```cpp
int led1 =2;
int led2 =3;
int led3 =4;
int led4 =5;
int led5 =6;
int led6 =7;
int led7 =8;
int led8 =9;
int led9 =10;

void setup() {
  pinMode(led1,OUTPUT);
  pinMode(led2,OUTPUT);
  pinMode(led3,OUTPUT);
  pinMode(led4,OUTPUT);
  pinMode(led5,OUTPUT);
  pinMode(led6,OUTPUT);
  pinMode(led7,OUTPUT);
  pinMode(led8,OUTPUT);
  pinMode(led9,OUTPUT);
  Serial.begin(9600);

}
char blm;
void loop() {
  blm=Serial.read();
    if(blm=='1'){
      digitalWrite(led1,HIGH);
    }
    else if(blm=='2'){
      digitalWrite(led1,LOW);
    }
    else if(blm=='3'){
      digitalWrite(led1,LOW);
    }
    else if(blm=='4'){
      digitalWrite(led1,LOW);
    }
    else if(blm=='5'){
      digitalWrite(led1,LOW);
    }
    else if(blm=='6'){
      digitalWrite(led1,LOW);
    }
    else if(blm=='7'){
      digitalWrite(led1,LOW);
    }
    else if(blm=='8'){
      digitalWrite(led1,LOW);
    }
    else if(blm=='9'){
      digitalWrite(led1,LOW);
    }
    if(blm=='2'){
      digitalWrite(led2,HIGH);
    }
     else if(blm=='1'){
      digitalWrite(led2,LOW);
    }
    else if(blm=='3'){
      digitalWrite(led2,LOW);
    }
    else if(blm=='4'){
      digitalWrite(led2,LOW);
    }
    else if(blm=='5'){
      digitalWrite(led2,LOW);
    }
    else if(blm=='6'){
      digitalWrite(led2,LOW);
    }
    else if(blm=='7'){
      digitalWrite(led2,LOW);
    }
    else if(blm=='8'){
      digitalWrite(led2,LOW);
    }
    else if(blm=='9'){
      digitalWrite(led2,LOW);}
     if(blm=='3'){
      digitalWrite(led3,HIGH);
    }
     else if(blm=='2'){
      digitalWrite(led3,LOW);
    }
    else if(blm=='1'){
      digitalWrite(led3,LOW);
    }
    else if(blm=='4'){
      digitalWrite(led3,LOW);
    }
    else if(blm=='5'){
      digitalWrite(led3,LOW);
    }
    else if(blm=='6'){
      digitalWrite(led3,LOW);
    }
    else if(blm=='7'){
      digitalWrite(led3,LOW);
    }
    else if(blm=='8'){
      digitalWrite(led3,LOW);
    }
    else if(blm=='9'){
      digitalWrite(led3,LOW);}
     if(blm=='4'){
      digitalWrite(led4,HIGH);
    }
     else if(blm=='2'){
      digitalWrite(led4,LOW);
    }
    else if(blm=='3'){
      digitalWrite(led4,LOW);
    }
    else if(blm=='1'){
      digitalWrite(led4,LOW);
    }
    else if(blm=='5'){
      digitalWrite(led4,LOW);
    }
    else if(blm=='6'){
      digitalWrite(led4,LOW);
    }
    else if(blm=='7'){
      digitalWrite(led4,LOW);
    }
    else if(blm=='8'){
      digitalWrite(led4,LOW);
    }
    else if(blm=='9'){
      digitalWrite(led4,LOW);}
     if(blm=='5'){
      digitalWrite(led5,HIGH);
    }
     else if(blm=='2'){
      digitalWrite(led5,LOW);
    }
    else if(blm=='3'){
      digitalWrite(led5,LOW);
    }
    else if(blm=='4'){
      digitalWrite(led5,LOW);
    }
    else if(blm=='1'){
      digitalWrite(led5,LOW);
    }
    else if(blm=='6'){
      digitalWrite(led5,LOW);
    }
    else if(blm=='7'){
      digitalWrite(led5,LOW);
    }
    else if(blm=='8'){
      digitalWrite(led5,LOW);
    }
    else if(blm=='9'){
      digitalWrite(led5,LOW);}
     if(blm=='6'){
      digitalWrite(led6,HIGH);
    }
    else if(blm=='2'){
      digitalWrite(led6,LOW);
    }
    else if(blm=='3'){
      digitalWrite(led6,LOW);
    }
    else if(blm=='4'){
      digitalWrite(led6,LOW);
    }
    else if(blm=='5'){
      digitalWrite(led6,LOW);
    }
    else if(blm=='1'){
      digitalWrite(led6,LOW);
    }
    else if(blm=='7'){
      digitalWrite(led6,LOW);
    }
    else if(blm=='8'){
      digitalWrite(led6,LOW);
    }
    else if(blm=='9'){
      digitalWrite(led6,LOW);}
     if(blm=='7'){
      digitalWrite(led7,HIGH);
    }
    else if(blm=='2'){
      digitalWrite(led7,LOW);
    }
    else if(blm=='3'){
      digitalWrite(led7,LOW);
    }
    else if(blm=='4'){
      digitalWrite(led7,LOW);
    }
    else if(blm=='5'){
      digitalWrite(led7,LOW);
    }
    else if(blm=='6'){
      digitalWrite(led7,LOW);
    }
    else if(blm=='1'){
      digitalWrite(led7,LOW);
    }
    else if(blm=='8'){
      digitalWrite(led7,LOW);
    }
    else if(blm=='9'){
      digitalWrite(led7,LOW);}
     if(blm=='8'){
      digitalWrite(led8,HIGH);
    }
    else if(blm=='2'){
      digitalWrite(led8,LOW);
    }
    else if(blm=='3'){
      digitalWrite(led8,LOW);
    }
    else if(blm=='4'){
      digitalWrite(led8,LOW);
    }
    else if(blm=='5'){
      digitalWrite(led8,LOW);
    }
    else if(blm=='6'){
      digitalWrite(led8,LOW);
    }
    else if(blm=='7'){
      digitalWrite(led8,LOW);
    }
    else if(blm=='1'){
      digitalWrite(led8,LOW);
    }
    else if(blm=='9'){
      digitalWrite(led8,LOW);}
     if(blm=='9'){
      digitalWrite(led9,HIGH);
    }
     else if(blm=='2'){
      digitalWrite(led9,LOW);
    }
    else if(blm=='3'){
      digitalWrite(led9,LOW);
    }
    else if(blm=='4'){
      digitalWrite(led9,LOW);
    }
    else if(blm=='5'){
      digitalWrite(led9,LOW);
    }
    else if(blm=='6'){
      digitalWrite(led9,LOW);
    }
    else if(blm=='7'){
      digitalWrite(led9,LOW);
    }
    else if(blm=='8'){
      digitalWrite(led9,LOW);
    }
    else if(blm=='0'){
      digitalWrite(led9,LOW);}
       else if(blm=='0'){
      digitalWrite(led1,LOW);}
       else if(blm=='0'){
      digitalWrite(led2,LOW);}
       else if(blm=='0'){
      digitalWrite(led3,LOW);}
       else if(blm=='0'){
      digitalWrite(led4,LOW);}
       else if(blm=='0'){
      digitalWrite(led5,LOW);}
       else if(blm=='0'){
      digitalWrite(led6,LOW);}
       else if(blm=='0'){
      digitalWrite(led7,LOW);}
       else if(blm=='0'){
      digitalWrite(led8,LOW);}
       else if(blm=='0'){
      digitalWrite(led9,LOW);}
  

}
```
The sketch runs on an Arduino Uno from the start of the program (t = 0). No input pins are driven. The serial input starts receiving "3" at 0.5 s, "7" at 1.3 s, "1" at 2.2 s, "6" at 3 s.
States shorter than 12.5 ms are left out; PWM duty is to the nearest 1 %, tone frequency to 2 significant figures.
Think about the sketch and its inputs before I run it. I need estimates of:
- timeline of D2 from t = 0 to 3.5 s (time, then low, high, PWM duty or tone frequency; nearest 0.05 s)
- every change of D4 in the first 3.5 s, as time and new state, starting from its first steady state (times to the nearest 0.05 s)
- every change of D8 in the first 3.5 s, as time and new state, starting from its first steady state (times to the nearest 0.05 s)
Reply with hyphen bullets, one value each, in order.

- 0 s low; 2.2 s high; 3 s low
- 0 s low; 0.5 s high; 1.3 s low
- 0 s low; 1.3 s high; 2.2 s low
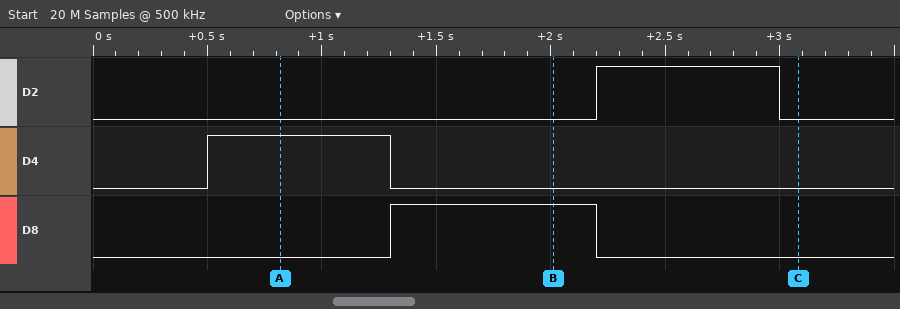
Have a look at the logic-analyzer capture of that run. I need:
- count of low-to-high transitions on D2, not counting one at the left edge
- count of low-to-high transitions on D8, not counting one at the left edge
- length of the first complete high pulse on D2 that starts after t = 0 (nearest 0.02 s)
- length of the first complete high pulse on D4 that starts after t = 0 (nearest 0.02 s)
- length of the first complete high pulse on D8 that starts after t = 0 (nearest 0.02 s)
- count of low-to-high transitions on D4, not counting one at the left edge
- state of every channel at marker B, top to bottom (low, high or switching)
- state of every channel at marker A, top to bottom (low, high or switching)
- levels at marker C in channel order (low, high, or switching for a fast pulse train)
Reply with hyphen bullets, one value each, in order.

- 1
- 1
- 0.80 s
- 0.80 s
- 0.90 s
- 1
- D2 low, D4 low, D8 high
- D2 low, D4 high, D8 low
- D2 low, D4 low, D8 low
